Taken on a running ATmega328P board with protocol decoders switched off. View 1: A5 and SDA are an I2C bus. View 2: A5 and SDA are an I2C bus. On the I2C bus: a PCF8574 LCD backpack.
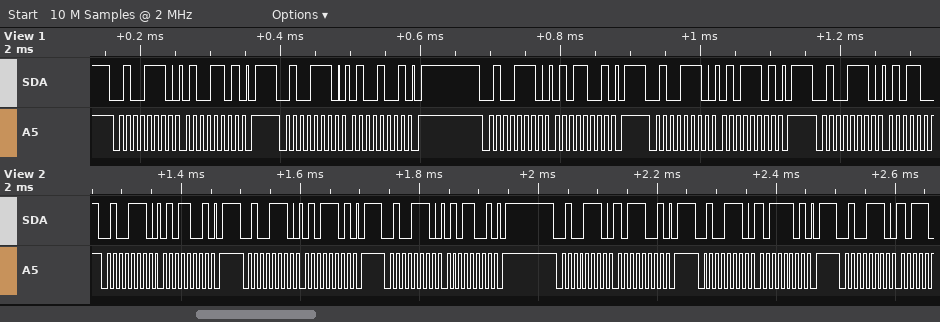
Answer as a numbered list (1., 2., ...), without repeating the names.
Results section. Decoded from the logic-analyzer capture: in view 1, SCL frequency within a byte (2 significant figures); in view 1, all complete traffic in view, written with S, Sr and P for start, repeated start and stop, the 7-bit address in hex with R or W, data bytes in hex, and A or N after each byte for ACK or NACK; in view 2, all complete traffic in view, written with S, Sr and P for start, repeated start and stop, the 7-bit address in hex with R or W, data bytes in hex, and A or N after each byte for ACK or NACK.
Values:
1. 100 kHz
2. S 27W A 4D A P S 27W A 49 A P S 27W A 59 A P S 27W A 5D A P S 27W A
3. S 27W A 59 A P S 27W A 5D A P S 27W A 59 A P S 27W A B9 A P S 27W A BD A P S 27W A
